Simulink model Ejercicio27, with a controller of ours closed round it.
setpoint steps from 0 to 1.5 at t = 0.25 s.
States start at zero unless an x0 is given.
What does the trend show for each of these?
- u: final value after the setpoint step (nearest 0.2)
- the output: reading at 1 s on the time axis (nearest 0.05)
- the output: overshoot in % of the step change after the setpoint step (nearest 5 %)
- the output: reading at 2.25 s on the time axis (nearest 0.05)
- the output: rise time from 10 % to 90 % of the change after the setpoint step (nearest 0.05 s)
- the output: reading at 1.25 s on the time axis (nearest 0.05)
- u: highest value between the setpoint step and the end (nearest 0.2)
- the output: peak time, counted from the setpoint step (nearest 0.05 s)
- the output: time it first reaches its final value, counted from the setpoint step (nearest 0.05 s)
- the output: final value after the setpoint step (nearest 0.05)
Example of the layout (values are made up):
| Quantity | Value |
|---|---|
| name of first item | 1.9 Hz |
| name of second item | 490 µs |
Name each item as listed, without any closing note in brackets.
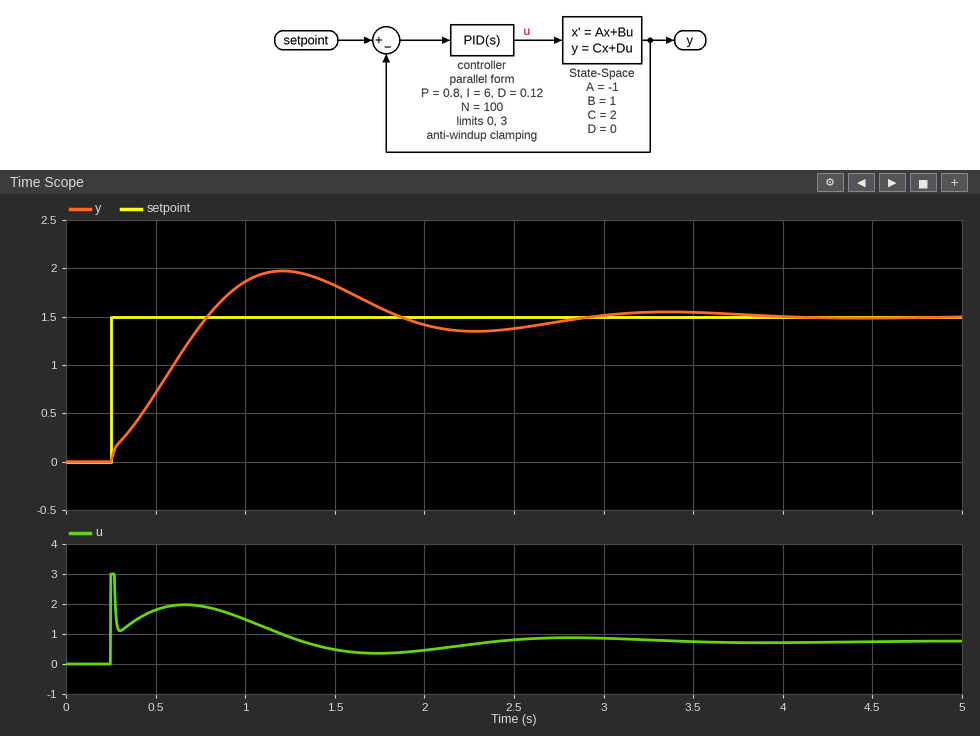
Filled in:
| Quantity | Value |
|---|---|
| u: final value after the setpoint step | 0.8 |
| the output: reading at 1 s on the time axis | 1.85 |
| the output: overshoot in % of the step change after the setpoint step | 30 % |
| the output: reading at 2.25 s on the time axis | 1.35 |
| the output: rise time from 10 % to 90 % of the change after the setpoint step | 0.45 s |
| the output: reading at 1.25 s on the time axis | 1.95 |
| u: highest value between the setpoint step and the end | 3.0 |
| the output: peak time, counted from the setpoint step | 0.95 s |
| the output: time it first reaches its final value, counted from the setpoint step | 0.55 s |
| the output: final value after the setpoint step | 1.50 |
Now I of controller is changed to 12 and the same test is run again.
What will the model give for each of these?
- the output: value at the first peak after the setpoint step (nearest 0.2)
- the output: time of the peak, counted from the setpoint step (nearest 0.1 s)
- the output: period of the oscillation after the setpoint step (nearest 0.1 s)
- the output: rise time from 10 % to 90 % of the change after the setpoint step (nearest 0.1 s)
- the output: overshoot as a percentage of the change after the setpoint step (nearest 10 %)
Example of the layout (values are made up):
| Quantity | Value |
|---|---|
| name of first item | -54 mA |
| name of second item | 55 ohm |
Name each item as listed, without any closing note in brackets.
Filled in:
| Quantity | Value |
|---|---|
| the output: value at the first peak after the setpoint step | 2.2 |
| the output: time of the peak, counted from the setpoint step | 0.7 s |
| the output: period of the oscillation after the setpoint step | 1.5 s |
| the output: rise time from 10 % to 90 % of the change after the setpoint step | 0.3 s |
| the output: overshoot as a percentage of the change after the setpoint step | 40 % |
